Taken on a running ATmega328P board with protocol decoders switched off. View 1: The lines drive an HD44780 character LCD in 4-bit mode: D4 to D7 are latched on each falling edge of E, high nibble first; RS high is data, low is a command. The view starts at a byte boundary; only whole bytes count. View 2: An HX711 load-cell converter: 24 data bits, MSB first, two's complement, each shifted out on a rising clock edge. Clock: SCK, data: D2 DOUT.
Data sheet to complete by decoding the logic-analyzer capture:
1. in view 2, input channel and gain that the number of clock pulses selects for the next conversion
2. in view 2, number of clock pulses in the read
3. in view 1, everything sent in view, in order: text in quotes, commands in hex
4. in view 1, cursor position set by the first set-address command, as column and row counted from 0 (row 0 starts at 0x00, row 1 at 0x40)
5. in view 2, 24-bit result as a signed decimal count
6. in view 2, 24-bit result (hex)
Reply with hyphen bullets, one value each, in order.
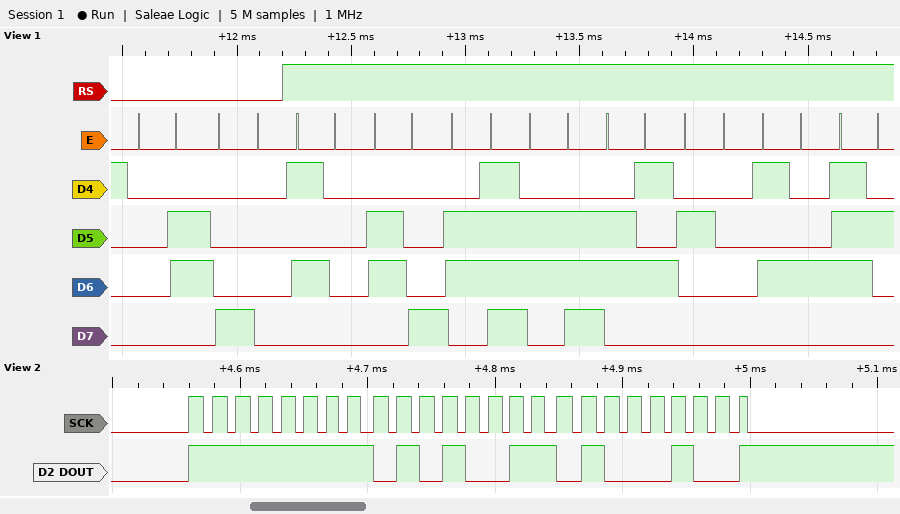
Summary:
- channel A, gain 128
- 25
- 0x06 0x80 "Phone Tr"
- column 0, row 0
- -44220
- 0xFF5344
